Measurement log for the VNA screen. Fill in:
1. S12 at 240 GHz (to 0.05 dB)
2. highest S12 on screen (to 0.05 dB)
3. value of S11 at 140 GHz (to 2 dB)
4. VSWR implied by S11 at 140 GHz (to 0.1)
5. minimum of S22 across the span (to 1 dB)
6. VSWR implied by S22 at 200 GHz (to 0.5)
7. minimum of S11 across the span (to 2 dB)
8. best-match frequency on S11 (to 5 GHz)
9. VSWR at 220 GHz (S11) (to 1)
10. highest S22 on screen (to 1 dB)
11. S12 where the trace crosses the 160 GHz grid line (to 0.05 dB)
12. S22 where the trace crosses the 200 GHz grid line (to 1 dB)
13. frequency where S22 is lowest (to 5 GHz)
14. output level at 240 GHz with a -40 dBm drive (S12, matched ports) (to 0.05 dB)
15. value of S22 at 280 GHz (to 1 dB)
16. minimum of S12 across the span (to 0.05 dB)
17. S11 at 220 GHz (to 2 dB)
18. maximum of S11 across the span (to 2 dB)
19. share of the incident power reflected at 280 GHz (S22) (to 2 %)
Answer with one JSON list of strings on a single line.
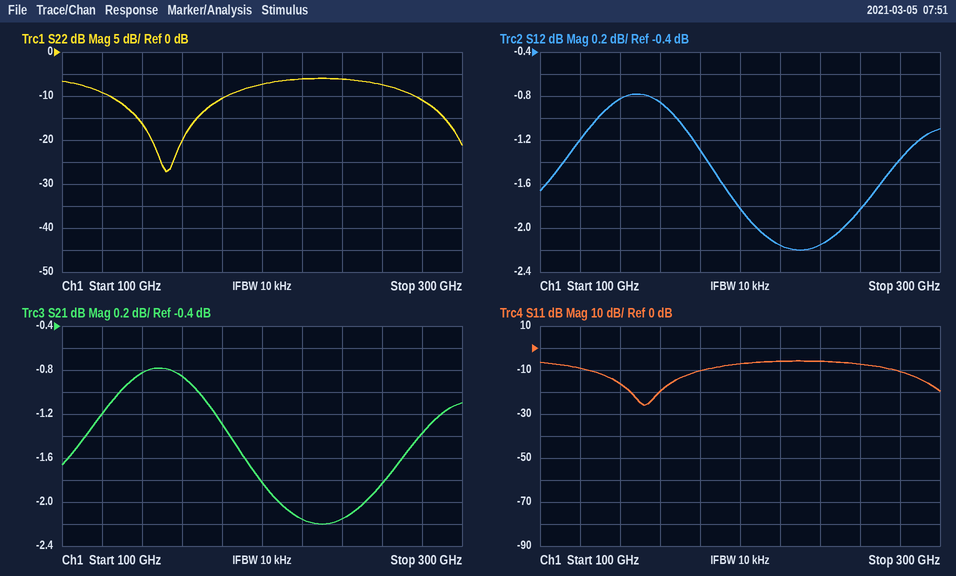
["-2.15 dB", "-0.80 dB", "-16 dB", "1.4", "-27 dB", "2.5", "-26 dB", "150 GHz", "3", "-6 dB", "-0.85 dB", "-7 dB", "150 GHz", "-42.15 dBm", "-11 dB", "-2.20 dB", "-6 dB", "-6 dB", "8 %"]
